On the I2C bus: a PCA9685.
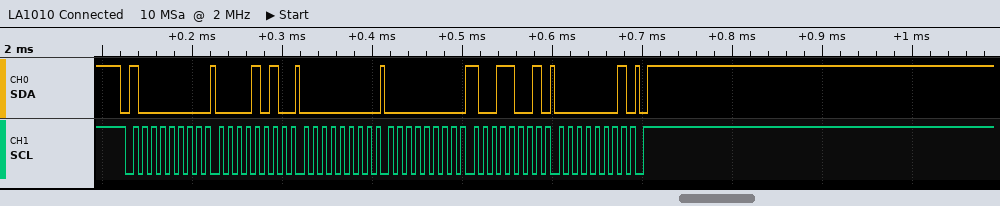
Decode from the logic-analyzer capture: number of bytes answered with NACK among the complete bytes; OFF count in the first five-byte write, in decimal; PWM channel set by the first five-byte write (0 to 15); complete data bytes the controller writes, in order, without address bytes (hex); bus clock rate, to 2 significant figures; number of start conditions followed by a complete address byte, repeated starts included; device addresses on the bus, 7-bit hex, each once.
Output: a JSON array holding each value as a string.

["0", "409", "1", "0A 00 00 99 01", "100 kHz", "1", "0x40"]
